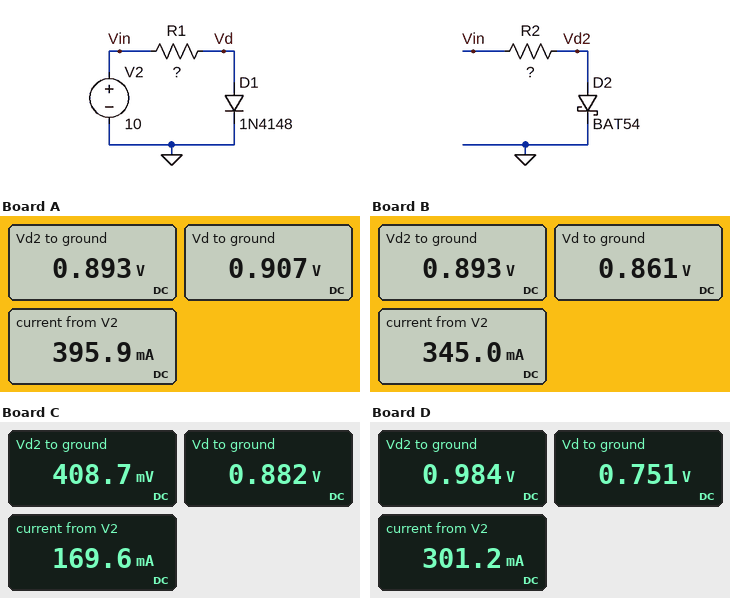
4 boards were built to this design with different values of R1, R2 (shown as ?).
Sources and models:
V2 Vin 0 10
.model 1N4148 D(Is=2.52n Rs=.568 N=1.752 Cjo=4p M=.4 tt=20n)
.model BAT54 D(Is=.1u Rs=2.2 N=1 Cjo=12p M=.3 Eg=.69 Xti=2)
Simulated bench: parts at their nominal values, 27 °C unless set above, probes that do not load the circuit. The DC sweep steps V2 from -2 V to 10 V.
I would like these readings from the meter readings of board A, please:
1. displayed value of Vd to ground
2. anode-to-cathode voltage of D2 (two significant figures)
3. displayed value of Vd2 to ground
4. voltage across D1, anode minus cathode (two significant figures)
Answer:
0.907 V
890 mV
0.893 V
910 mV
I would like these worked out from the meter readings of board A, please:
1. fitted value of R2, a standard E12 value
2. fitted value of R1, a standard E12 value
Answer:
39 Ω
56 Ω
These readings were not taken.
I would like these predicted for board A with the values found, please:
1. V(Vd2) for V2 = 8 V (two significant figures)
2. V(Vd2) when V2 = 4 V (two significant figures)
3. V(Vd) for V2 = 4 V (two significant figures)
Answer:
780 mV
550 mV
800 mV
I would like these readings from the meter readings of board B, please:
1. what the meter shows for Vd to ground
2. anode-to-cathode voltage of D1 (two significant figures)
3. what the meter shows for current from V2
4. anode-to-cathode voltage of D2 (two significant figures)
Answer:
0.861 V
860 mV
345.0 mA
890 mV
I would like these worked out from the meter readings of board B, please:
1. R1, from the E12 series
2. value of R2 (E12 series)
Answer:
82 Ω
39 Ω
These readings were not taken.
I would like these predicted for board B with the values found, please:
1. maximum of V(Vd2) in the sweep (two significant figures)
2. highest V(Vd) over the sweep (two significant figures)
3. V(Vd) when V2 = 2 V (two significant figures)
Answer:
890 mV
860 mV
720 mV
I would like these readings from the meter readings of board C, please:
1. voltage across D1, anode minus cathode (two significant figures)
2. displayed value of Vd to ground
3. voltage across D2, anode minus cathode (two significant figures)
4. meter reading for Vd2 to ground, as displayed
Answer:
880 mV
0.882 V
410 mV
408.7 mV
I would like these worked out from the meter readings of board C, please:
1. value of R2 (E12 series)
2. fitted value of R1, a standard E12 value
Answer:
270 Ω
68 Ω
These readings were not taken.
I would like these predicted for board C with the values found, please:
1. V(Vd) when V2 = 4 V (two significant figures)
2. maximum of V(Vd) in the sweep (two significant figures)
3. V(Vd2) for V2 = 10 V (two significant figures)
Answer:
790 mV
880 mV
410 mV
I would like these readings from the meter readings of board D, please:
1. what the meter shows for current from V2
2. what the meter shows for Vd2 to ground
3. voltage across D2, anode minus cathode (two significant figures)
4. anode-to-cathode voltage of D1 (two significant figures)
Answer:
301.2 mA
0.984 V
980 mV
750 mV
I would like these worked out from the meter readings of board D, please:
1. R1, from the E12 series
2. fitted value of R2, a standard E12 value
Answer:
330 Ω
33 Ω
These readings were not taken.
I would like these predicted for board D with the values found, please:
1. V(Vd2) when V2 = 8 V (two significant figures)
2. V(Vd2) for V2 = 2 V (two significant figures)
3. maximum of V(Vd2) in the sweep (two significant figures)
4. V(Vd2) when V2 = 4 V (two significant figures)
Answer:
850 mV
440 mV
980 mV
590 mV
